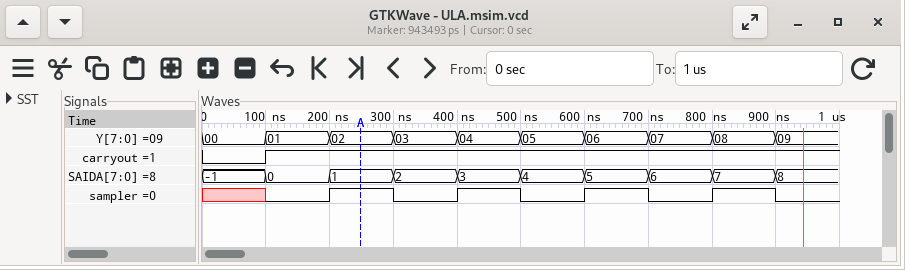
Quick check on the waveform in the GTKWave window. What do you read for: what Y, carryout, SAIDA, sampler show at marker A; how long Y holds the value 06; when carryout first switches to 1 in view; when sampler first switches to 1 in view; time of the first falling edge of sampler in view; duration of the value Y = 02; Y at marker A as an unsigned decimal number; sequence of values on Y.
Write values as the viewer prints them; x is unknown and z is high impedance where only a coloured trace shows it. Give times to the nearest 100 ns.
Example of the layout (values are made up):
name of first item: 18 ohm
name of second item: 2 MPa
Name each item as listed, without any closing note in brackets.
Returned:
what Y, carryout, SAIDA, sampler show at marker A: Y=02, carryout=1, SAIDA=1, sampler=1
how long Y holds the value 06: 100 ns
when carryout first switches to 1 in view: 100 ns
when sampler first switches to 1 in view: 200 ns
time of the first falling edge of sampler in view: 300 ns
duration of the value Y = 02: 100 ns
Y at marker A as an unsigned decimal number: 2
sequence of values on Y: 00, 01, 02, 03, 04, 05, 06, 07, 08, 09
